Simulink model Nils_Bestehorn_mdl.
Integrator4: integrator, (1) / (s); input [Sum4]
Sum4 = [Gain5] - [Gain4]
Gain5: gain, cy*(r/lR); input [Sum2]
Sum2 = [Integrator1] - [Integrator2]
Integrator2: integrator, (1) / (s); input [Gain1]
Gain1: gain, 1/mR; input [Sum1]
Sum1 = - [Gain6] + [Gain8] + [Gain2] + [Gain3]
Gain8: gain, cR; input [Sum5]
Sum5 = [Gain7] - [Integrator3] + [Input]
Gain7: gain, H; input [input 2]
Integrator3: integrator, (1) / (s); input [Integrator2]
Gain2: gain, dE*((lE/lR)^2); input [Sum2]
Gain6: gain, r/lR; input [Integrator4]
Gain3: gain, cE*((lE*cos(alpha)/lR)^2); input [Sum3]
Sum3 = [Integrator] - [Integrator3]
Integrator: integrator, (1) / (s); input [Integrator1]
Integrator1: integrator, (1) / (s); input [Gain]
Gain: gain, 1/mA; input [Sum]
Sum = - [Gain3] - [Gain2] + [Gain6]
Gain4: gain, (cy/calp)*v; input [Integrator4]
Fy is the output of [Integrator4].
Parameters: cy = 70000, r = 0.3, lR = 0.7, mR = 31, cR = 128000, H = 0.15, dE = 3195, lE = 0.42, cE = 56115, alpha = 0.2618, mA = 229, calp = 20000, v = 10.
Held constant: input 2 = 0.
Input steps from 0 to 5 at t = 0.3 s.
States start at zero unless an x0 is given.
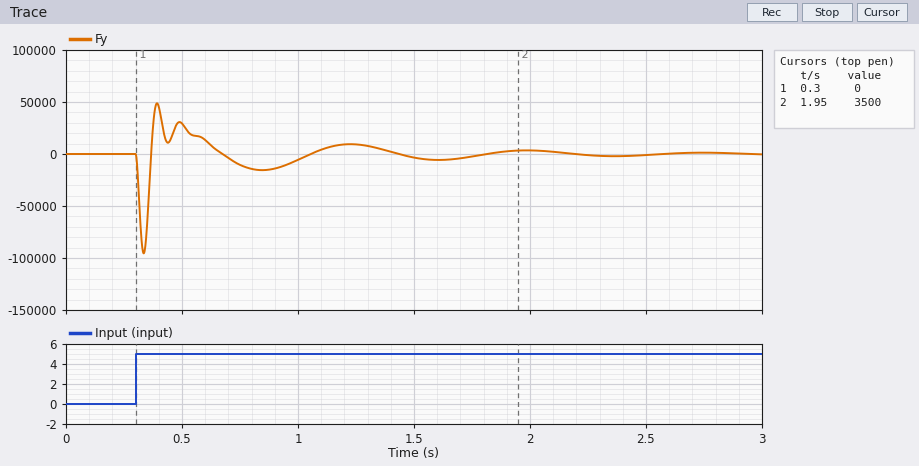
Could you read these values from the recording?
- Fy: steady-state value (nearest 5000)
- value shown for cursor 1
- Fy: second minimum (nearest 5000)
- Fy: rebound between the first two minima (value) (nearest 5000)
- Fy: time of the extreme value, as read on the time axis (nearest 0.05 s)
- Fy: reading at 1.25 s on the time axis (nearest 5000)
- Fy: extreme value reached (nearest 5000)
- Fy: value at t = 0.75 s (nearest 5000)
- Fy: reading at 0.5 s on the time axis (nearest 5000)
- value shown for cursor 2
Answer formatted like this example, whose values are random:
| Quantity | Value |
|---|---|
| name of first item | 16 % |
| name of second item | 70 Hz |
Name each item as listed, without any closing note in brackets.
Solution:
| Quantity | Value |
|---|---|
| Fy: steady-state value | 0 |
| value shown for cursor 1 | 0 |
| Fy: second minimum | 10000 |
| Fy: rebound between the first two minima (value) | 50000 |
| Fy: time of the extreme value, as read on the time axis | 0.35 s |
| Fy: reading at 1.25 s on the time axis | 10000 |
| Fy: extreme value reached | -95000 |
| Fy: value at t = 0.75 s | -10000 |
| Fy: reading at 0.5 s on the time axis | 30000 |
| value shown for cursor 2 | 3500 |
